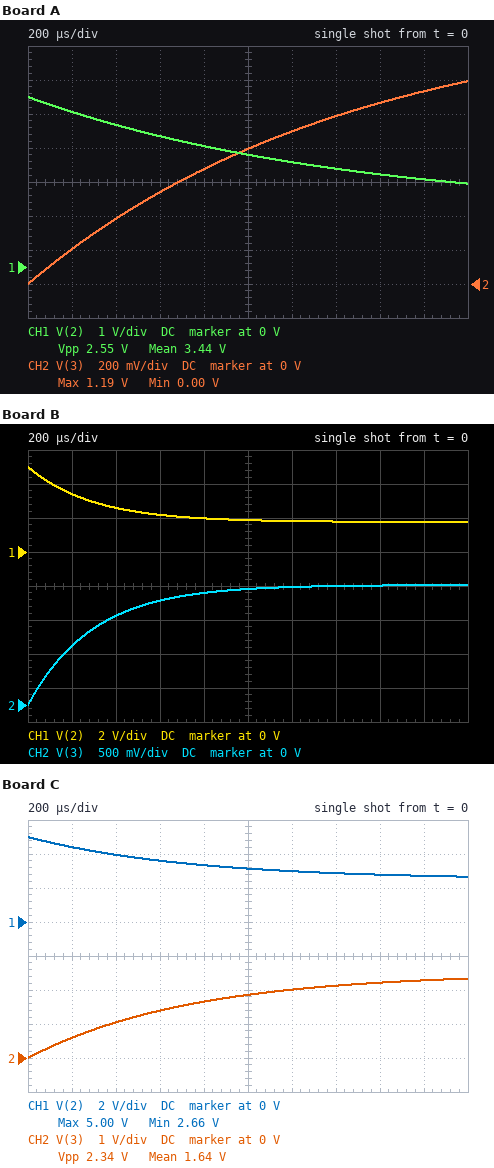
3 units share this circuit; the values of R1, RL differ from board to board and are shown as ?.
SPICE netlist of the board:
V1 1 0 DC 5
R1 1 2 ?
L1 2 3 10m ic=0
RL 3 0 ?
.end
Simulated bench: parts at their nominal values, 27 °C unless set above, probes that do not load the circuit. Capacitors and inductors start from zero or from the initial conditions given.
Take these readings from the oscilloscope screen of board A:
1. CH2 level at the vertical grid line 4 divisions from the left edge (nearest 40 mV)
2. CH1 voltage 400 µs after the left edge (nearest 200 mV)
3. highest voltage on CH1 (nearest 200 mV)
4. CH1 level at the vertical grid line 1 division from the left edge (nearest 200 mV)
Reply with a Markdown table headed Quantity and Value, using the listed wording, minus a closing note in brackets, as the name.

| Quantity | Value |
|---|---|
| CH2 level at the vertical grid line 4 divisions from the left edge | 680 mV |
| CH1 voltage 400 µs after the left edge | 4.2 V |
| highest voltage on CH1 | 5.0 V |
| CH1 level at the vertical grid line 1 division from the left edge | 4.6 V |
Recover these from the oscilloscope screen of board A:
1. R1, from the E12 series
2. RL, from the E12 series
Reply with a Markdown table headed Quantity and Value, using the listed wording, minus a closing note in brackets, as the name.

| Quantity | Value |
|---|---|
| R1, from the E12 series | 4.7 Ω |
| RL, from the E12 series | 2.2 Ω |
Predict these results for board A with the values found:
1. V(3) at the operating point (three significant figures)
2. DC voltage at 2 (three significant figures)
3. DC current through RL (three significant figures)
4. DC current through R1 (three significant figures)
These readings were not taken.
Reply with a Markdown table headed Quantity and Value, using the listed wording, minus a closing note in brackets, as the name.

| Quantity | Value |
|---|---|
| V(3) at the operating point | 1.59 V |
| DC voltage at 2 | 1.59 V |
| DC current through RL | 725 mA |
| DC current through R1 | 725 mA |
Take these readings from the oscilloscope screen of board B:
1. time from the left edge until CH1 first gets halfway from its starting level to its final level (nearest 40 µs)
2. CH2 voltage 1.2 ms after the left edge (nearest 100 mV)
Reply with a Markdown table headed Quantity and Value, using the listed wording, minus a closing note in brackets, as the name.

| Quantity | Value |
|---|---|
| time from the left edge until CH1 first gets halfway from its starting level to its final level | 200 µs |
| CH2 voltage 1.2 ms after the left edge | 1.7 V |
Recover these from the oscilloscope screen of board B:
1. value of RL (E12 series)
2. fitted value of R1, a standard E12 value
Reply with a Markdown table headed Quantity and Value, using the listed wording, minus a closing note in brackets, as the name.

| Quantity | Value |
|---|---|
| value of RL | 12 Ω |
| fitted value of R1, a standard E12 value | 22 Ω |
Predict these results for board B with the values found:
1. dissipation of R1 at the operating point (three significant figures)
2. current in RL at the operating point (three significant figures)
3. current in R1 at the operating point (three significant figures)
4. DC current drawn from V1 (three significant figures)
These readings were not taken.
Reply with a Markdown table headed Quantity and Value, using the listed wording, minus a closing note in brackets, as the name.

| Quantity | Value |
|---|---|
| dissipation of R1 at the operating point | 476 mW |
| current in RL at the operating point | 147 mA |
| current in R1 at the operating point | 147 mA |
| DC current drawn from V1 | 147 mA |
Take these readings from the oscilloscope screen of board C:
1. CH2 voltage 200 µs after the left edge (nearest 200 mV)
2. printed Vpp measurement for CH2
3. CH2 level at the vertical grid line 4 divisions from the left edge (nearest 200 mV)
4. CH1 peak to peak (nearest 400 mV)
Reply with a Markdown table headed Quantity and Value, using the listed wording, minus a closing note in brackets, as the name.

| Quantity | Value |
|---|---|
| CH2 voltage 200 µs after the left edge | 600 mV |
| printed Vpp measurement for CH2 | 2.34 V |
| CH2 level at the vertical grid line 4 divisions from the left edge | 1.6 V |
| CH1 peak to peak | 2.4 V |
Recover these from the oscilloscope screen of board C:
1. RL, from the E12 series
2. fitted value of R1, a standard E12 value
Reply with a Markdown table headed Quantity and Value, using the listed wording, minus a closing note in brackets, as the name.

| Quantity | Value |
|---|---|
| RL, from the E12 series | 6.8 Ω |
| fitted value of R1, a standard E12 value | 6.8 Ω |
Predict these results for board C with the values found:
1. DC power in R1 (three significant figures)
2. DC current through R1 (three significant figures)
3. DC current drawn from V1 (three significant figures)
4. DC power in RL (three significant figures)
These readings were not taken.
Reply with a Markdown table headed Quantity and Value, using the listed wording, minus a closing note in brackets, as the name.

| Quantity | Value |
|---|---|
| DC power in R1 | 919 mW |
| DC current through R1 | 368 mA |
| DC current drawn from V1 | 368 mA |
| DC power in RL | 919 mW |
